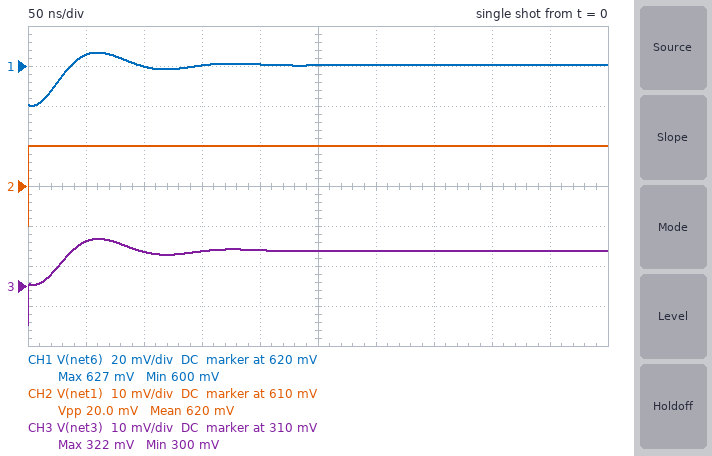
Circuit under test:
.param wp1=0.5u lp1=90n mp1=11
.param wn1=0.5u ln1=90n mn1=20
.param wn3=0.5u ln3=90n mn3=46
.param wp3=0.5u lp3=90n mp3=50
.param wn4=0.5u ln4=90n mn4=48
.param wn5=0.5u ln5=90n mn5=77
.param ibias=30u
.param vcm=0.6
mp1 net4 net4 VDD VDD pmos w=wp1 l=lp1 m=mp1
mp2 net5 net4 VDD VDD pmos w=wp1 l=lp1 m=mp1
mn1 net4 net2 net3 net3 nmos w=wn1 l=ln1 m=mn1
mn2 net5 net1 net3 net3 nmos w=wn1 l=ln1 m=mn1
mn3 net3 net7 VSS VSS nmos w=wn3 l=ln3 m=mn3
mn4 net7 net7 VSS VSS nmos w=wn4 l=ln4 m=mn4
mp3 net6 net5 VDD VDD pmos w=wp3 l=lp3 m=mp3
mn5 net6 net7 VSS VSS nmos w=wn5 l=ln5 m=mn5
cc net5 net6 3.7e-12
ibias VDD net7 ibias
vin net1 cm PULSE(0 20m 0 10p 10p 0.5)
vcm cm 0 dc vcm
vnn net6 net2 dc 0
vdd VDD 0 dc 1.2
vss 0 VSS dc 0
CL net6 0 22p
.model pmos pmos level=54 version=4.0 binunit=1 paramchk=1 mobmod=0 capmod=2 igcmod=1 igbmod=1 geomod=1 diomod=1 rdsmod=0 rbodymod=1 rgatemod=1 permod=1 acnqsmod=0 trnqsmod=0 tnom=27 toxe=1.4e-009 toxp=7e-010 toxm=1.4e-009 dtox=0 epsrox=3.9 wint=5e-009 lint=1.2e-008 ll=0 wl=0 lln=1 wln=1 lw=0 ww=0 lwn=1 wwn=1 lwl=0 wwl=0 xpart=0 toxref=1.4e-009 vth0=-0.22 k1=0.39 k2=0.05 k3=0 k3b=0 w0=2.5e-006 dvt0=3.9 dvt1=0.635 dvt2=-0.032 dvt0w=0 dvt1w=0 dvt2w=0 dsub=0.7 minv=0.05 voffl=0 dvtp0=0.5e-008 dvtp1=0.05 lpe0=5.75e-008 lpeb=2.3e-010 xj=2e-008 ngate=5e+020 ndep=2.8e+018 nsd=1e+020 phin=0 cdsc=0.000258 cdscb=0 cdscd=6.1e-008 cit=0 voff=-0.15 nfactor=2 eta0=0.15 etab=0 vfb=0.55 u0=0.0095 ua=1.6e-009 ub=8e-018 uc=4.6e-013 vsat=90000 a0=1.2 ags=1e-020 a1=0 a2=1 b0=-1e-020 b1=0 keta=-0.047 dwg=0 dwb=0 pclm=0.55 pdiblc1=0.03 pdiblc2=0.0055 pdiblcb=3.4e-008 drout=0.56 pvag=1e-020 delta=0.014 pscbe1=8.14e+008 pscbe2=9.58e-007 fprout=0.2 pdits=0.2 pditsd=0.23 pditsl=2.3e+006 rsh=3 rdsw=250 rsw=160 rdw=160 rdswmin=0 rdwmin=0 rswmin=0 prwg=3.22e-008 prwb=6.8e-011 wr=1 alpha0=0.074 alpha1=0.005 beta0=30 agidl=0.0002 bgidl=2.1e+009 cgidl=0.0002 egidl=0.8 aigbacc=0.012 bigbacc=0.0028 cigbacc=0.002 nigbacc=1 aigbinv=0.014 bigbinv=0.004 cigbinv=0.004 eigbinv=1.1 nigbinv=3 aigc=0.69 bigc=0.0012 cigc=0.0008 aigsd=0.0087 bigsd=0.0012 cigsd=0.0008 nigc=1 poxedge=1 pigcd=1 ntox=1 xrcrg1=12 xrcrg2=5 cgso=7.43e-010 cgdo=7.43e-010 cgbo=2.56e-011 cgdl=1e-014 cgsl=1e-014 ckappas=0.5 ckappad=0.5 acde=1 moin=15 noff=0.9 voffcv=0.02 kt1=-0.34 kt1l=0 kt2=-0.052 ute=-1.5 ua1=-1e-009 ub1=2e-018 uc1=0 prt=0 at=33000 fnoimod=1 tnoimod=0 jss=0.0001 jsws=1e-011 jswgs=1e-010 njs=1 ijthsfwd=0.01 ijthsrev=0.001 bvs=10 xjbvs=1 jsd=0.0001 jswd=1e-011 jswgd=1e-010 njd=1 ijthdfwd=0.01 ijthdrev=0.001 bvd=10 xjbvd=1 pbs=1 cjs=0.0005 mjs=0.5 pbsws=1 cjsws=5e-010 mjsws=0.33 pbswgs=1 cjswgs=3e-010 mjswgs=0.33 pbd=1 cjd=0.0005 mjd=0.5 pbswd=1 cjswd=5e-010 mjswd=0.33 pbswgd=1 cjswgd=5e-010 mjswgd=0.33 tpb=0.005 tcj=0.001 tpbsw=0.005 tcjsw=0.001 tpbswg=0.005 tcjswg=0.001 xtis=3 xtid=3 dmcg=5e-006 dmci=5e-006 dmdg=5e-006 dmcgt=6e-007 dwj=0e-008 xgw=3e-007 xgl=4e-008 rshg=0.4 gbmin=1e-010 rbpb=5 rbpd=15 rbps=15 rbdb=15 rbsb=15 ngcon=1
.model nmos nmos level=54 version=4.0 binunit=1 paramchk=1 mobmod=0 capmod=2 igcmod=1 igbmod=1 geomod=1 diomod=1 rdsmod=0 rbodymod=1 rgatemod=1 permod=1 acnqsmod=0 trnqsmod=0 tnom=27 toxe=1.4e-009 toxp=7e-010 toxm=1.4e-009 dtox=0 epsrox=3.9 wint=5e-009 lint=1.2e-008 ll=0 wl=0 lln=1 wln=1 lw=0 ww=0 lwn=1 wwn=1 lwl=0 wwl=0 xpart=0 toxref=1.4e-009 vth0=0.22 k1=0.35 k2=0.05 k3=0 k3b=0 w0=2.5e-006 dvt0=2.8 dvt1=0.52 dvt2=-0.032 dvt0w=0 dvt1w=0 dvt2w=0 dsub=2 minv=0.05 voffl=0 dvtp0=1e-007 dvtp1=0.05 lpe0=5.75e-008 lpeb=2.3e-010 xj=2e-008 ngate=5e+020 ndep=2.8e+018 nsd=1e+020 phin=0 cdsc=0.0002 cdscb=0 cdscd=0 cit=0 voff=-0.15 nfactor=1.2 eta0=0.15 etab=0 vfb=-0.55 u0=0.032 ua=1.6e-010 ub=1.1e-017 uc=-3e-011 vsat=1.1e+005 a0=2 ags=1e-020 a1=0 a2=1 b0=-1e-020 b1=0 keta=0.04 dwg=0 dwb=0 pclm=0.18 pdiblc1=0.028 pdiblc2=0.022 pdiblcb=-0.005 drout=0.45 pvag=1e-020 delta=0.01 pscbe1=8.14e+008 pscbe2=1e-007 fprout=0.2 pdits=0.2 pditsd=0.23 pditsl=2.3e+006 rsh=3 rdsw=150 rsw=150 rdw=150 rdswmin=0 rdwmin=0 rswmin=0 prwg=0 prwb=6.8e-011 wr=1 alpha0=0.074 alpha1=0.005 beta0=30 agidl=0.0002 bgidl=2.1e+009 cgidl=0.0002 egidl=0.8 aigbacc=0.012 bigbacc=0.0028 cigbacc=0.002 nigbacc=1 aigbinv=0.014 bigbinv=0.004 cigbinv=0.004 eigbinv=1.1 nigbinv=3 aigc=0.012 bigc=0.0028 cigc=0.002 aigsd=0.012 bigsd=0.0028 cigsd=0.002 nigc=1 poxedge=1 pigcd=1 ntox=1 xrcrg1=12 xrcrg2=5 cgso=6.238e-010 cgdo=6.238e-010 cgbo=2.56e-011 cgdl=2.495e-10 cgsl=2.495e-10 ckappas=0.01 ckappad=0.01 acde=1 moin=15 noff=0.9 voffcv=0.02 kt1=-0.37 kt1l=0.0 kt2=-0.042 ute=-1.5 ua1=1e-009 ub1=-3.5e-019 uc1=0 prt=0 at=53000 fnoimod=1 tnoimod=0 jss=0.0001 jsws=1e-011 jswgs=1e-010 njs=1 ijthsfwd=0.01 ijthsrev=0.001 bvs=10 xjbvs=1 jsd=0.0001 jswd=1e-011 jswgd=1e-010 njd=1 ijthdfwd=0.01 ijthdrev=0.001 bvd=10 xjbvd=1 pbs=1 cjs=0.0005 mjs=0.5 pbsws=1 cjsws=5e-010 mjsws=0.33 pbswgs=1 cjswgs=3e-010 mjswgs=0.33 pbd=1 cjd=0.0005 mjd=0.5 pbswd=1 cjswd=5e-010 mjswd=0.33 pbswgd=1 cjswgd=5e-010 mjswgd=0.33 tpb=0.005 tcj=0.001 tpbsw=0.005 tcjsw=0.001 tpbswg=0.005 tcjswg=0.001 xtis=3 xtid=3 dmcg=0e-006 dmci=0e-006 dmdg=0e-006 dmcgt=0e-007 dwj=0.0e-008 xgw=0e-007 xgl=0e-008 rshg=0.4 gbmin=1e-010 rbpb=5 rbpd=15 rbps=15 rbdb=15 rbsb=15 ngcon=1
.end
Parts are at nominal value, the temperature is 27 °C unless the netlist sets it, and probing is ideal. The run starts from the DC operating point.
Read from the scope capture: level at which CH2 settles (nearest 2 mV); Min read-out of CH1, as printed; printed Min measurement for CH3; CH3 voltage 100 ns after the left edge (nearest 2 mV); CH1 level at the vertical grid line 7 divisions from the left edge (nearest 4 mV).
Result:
620 mV
600 mV
300 mV
318 mV
620 mV
